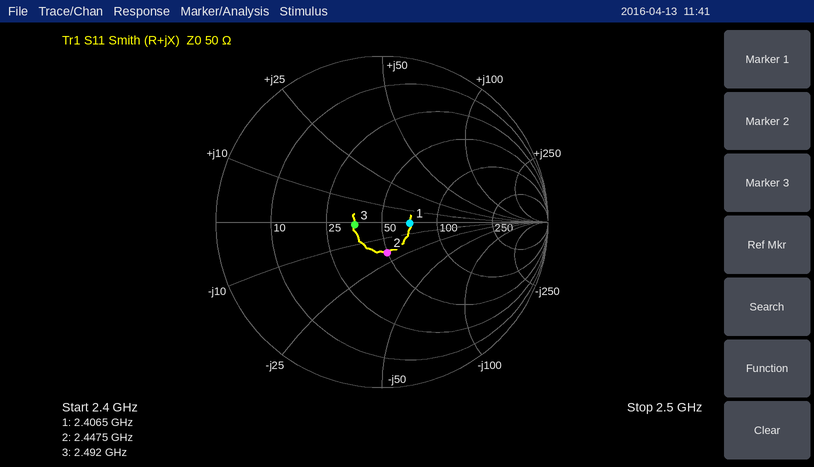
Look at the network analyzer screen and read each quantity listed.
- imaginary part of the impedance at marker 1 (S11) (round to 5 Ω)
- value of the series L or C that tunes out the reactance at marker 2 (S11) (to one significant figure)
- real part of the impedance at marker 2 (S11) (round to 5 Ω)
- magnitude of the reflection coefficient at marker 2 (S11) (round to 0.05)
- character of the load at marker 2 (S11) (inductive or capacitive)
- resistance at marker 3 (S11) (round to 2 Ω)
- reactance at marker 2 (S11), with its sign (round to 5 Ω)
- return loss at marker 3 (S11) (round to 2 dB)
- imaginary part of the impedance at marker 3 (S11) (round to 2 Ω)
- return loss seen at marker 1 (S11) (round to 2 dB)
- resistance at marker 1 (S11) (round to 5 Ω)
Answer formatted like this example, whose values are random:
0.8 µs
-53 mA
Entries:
0 Ω
1 nH
50 Ω
0.20
capacitive
36 Ω
-20 Ω
16 dB
-2 Ω
16 dB
70 Ω
